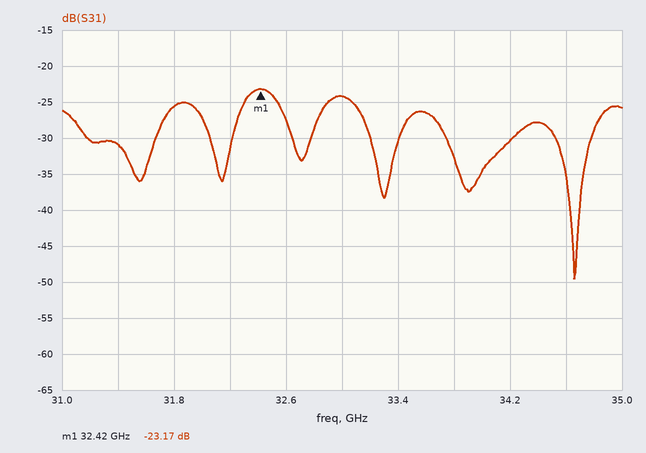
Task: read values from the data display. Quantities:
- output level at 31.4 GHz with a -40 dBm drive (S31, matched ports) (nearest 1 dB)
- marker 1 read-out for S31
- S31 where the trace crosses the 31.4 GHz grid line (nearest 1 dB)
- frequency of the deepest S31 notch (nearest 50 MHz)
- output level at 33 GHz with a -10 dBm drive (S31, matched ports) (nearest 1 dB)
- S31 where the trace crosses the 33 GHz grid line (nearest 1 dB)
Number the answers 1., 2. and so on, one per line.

1. -71 dBm
2. -23.17 dB
3. -31 dB
4. 34.65 GHz
5. -34 dBm
6. -24 dB
